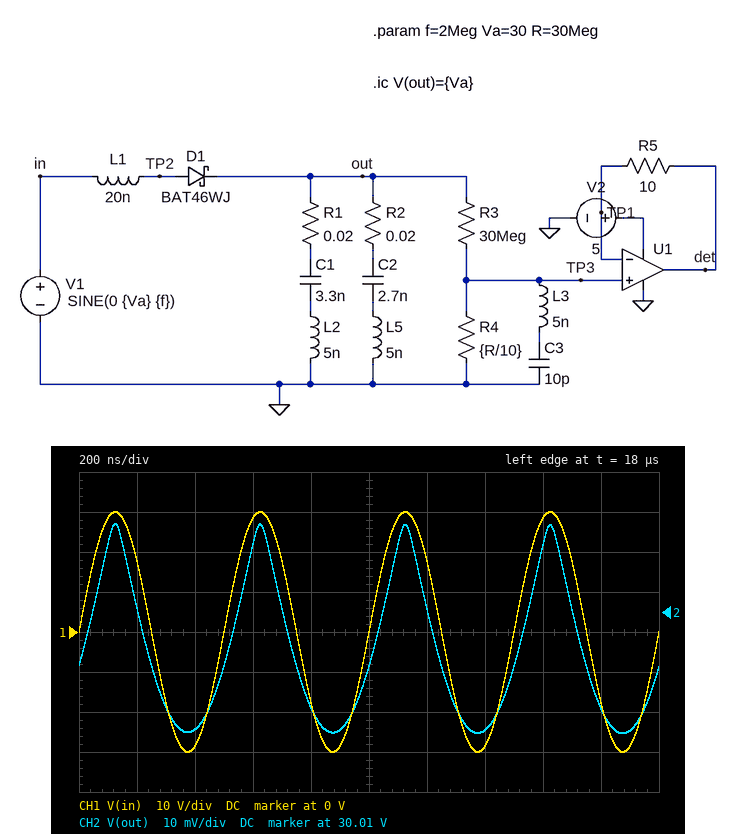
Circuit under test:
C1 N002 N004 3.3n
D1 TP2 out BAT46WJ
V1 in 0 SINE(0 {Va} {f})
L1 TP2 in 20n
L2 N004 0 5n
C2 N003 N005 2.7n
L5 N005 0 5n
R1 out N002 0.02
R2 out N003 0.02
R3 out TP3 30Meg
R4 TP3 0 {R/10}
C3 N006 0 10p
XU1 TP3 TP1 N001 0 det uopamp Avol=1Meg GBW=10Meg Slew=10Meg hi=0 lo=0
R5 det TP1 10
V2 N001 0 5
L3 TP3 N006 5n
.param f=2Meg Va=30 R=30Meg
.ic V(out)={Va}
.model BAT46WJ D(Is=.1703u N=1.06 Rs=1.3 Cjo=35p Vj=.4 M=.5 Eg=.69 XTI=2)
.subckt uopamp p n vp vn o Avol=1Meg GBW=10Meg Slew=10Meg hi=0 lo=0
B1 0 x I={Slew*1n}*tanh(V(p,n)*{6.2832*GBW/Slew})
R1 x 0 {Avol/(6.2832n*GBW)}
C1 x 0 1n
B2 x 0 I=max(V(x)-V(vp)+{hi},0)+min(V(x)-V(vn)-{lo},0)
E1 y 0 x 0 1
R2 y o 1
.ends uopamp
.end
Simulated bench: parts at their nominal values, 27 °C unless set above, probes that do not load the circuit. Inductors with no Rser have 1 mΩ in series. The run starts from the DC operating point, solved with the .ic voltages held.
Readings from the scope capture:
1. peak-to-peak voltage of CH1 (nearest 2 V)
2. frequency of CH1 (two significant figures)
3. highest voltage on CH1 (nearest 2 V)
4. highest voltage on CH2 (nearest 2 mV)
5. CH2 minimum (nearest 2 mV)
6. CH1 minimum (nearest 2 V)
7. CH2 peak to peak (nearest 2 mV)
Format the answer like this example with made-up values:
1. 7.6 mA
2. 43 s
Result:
1. 60 V
2. 2.0 MHz
3. 30 V
4. 30.032 V
5. 29.980 V
6. -30 V
7. 52 mV
